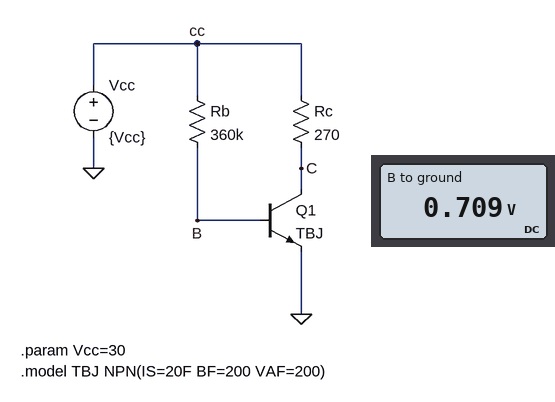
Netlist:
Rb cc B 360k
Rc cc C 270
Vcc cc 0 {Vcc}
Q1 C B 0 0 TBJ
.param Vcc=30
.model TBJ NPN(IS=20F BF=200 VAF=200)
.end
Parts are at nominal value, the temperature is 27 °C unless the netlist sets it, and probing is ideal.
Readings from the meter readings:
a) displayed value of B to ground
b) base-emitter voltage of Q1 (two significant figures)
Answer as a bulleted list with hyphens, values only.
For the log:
- 0.709 V
- 710 mV
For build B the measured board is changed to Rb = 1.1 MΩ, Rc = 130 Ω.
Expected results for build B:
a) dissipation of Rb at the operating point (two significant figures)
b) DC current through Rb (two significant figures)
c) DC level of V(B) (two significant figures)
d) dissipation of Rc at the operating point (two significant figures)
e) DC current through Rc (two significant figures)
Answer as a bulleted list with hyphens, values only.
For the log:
- 780 µW
- 27 µA
- 680 mV
- 4.8 mW
- 6.1 mA
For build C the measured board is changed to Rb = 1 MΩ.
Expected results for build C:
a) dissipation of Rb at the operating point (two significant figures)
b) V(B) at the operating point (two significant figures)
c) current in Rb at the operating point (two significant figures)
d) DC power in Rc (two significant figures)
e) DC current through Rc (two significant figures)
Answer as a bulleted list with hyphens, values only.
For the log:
- 860 µW
- 680 mV
- 29 µA
- 12 mW
- 6.7 mA
